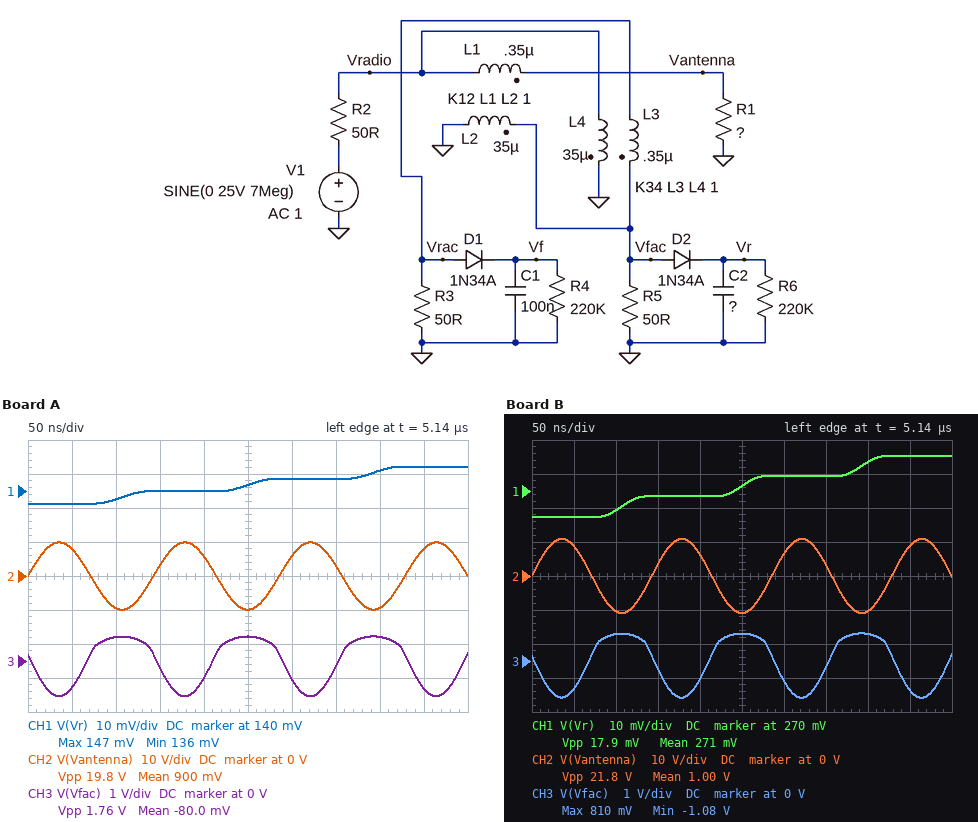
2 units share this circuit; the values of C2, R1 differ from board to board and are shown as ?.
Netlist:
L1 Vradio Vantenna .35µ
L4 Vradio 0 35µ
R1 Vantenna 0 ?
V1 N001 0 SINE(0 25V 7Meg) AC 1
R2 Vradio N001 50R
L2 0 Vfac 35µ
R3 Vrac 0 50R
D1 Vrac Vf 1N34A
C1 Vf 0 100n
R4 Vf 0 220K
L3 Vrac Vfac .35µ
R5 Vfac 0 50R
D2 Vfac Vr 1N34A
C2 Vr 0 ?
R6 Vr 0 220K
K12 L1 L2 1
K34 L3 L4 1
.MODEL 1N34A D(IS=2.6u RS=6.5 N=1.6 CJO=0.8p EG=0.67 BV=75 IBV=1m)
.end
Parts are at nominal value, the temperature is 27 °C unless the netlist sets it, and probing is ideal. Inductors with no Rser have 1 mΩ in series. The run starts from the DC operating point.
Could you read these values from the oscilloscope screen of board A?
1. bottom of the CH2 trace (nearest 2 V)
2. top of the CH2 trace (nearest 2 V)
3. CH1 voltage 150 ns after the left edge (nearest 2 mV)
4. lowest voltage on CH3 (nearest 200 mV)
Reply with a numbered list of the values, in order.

1. -10 V
2. 10 V
3. 140 mV
4. -1.0 V
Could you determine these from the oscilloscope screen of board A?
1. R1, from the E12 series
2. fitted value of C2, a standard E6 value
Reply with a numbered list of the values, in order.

1. 33 Ω
2. 330 nF
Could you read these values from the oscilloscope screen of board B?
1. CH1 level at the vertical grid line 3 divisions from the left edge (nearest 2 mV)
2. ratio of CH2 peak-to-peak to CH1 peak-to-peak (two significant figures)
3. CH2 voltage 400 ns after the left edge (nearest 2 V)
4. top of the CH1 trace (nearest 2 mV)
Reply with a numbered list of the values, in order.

1. 268 mV
2. 1200
3. -10 V
4. 280 mV
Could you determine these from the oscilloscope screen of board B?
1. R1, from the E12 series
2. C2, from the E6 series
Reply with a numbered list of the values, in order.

1. 39 Ω
2. 150 nF
